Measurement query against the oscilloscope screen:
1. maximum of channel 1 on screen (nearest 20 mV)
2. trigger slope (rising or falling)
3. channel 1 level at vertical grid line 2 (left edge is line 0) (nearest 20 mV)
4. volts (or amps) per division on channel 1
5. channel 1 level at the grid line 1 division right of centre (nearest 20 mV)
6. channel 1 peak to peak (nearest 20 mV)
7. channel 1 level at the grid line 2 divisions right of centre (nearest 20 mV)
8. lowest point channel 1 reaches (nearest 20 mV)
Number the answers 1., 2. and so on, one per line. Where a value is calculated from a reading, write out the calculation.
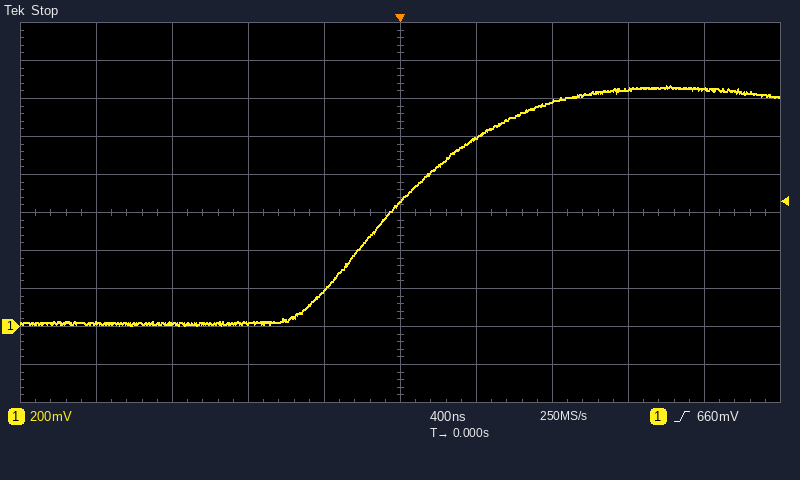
1. 1.26 V
2. rising
3. 20 mV
4. 200 mV
5. 1.00 V
6. 1.26 V − (0 mV) = 1.26 V
7. 1.18 V
8. 0 mV
